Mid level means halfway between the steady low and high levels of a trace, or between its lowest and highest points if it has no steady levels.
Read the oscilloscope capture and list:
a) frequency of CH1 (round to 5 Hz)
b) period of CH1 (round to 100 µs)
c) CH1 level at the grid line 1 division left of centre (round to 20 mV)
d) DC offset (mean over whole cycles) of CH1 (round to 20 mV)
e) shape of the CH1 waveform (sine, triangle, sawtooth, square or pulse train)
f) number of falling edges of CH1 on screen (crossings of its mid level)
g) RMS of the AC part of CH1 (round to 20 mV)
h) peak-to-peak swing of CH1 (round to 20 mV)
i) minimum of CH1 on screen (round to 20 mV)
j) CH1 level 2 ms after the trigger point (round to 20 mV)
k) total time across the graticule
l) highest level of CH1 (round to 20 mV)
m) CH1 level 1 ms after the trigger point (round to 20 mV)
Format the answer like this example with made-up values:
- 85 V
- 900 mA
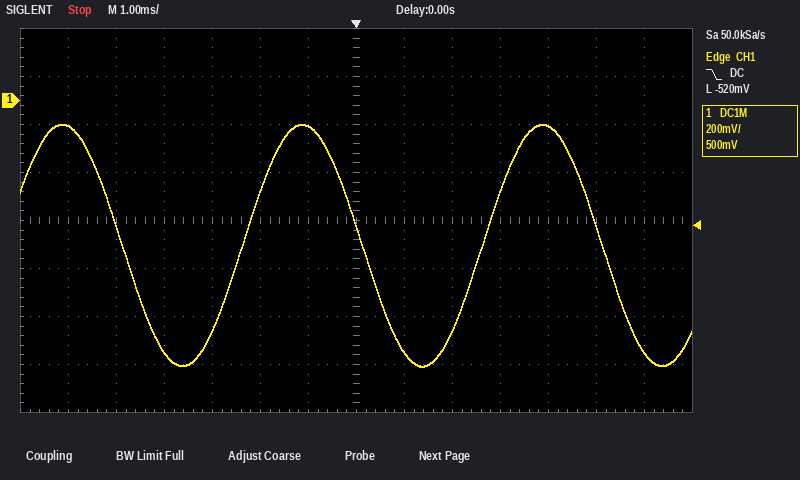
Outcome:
- 200 Hz
- 5.0 ms
- -100 mV
- -600 mV
- sine
- 3
- 360 mV
- 1.00 V
- -1.10 V
- -960 mV
- 14 ms
- -100 mV
- -1.04 V
